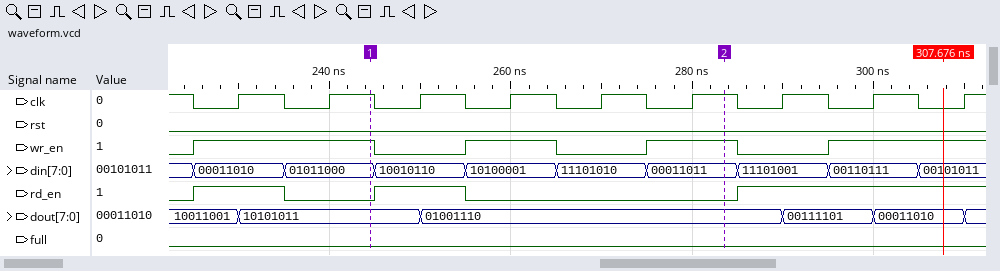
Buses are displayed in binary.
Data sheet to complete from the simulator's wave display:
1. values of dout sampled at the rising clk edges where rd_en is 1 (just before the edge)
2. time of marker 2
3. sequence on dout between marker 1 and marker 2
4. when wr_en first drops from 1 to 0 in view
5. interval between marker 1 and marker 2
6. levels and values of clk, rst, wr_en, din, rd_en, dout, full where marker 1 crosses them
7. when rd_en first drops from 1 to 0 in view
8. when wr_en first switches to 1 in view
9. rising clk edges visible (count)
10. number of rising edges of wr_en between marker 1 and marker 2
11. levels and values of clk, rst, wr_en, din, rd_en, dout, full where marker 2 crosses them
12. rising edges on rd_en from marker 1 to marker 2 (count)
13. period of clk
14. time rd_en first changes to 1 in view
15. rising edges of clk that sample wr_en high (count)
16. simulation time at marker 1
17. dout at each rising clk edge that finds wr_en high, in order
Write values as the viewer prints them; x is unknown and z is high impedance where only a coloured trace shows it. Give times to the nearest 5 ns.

10011001, 10101011, 01001110, 00111101, 00011010
285 ns
10101011, 01001110
245 ns
40 ns
clk=1, rst=0, wr_en=1, din=01011000, rd_en=0, dout=10101011, full=0
235 ns
225 ns
9
2
clk=1, rst=0, wr_en=1, din=00011011, rd_en=0, dout=01001110, full=0
1
10 ns
225 ns
6
245 ns
10011001, 10101011, 01001110, 01001110, 00111101, 00011010
